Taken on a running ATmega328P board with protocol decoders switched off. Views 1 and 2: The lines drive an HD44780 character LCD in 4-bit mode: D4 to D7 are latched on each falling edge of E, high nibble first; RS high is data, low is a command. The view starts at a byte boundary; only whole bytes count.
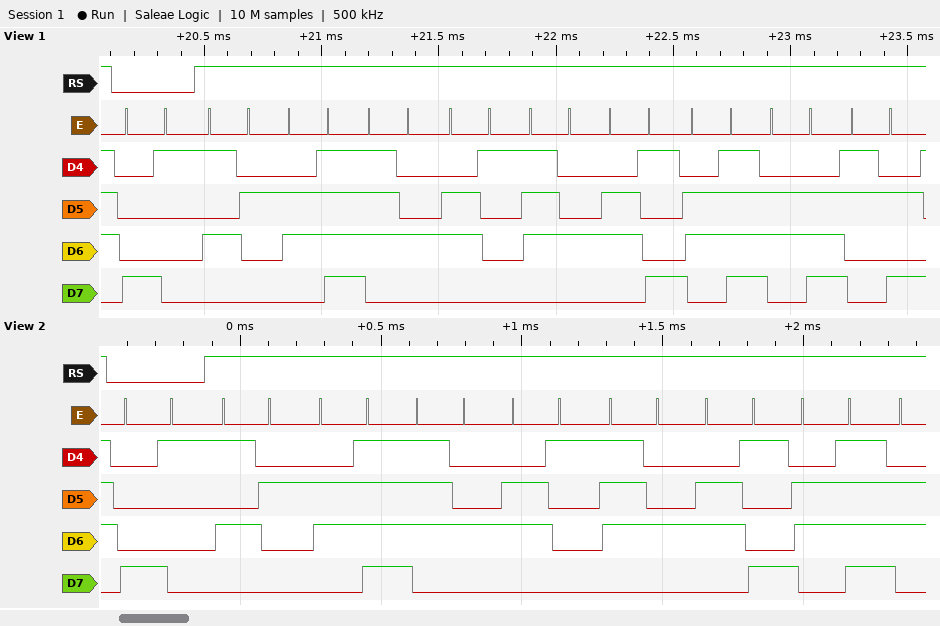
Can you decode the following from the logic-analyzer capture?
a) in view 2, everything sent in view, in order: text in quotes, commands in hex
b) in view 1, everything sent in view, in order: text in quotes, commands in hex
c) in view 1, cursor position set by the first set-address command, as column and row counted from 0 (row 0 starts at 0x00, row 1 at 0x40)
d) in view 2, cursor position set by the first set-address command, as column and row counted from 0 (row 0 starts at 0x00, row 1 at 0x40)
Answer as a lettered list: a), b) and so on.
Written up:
a) 0x81 "Rotatio"
b) 0x81 "Rotation:"
c) column 1, row 0
d) column 1, row 0
